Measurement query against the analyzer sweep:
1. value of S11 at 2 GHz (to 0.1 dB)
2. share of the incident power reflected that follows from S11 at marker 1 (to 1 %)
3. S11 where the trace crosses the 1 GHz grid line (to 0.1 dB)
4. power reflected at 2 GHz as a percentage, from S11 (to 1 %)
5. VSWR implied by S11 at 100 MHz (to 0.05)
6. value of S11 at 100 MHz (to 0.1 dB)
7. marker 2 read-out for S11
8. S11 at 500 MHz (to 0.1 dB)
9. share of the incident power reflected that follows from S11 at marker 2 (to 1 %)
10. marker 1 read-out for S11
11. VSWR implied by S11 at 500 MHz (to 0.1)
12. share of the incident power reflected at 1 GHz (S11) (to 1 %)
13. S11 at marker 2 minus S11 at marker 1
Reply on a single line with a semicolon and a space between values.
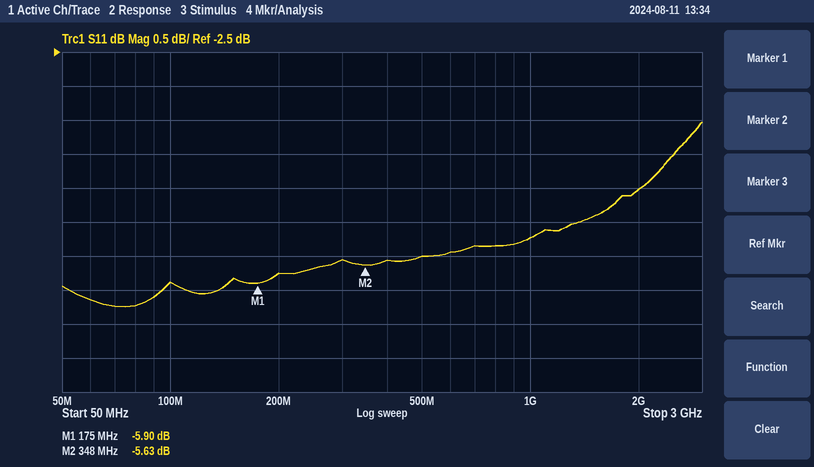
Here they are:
-4.5 dB; 26 %; -5.2 dB; 35 %; 3.05; -5.9 dB; -5.63 dB; -5.5 dB; 27 %; -5.90 dB; 3.3; 30 %; 0.27 dB
